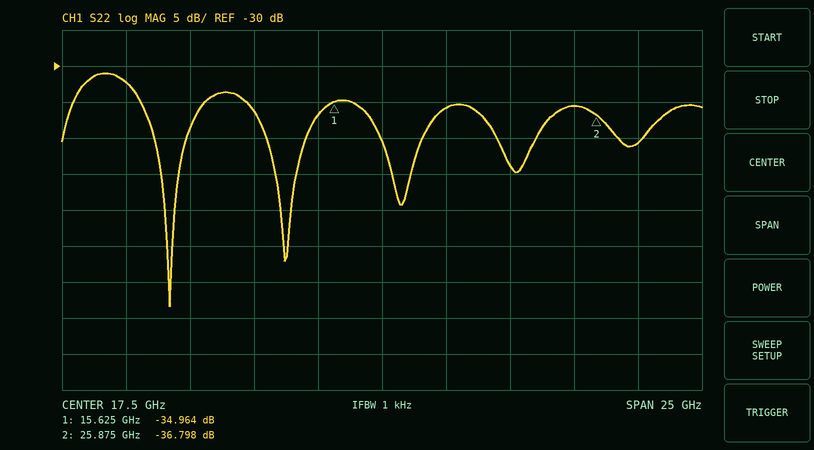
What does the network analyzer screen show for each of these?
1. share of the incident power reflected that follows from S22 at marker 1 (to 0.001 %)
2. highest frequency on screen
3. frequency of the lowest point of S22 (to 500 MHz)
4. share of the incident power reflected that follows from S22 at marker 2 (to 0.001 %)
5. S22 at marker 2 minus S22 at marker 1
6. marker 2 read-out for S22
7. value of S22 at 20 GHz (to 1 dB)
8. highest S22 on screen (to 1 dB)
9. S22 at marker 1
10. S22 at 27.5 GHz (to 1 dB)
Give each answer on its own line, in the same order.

0.032 %
30 GHz
9.0 GHz
0.021 %
-1.834 dB
-36.798 dB
-36 dB
-31 dB
-34.964 dB
-41 dB
